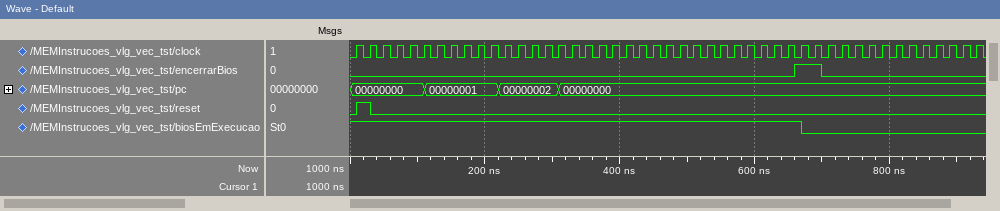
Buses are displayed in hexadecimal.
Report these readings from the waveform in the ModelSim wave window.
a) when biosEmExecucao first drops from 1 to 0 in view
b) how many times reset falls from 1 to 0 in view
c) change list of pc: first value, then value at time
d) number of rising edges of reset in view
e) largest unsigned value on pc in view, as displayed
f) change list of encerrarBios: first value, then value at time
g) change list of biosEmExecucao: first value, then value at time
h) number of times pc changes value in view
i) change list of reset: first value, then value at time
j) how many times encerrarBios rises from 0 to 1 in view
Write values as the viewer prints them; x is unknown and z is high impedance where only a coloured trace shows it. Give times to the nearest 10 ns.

670 ns
1
00000000, 00000001 at 110 ns, 00000002 at 220 ns, 00000000 at 310 ns
1
00000002
0, 1 at 660 ns, 0 at 700 ns
1, 0 at 670 ns
3
0, 1 at 10 ns, 0 at 30 ns
1
